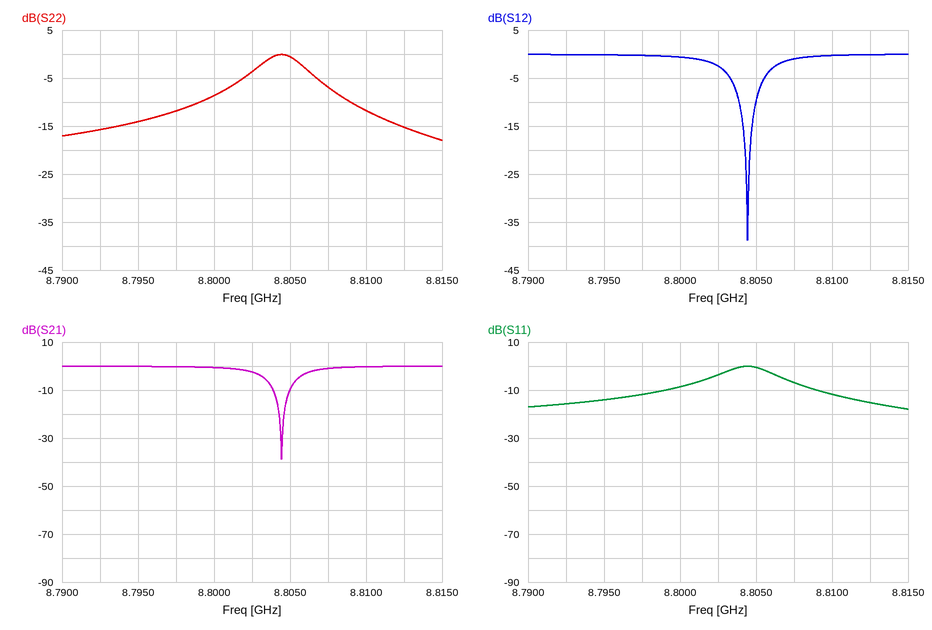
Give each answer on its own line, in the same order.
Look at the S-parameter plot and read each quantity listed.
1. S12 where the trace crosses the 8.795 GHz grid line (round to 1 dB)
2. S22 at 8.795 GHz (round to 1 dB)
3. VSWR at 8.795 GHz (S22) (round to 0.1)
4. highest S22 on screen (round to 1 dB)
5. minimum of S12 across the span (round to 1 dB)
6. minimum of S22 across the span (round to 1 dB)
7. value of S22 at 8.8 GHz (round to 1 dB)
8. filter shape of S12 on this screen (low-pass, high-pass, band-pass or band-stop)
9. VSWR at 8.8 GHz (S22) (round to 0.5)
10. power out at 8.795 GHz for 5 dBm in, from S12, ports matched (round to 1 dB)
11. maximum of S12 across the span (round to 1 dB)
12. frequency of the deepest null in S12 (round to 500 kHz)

0 dB
-14 dB
1.5
0 dB
-39 dB
-18 dB
-9 dB
band-stop
2.0
5 dBm
0 dB
8.8045 GHz
